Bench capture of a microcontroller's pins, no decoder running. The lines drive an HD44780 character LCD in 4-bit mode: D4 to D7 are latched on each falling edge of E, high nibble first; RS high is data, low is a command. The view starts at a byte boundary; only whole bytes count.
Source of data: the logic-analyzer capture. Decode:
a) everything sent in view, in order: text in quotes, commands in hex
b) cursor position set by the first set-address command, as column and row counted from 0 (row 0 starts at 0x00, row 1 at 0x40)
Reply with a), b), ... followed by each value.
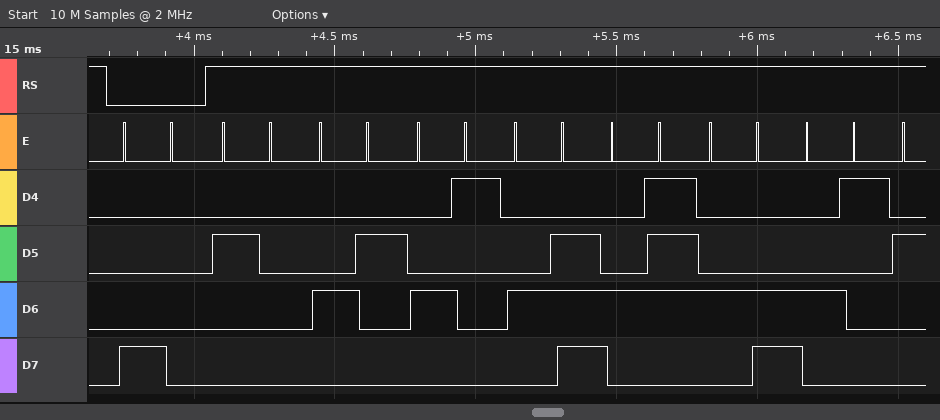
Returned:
a) 0x80 " BANGLA"
b) column 0, row 0
